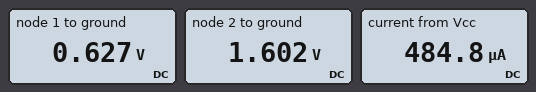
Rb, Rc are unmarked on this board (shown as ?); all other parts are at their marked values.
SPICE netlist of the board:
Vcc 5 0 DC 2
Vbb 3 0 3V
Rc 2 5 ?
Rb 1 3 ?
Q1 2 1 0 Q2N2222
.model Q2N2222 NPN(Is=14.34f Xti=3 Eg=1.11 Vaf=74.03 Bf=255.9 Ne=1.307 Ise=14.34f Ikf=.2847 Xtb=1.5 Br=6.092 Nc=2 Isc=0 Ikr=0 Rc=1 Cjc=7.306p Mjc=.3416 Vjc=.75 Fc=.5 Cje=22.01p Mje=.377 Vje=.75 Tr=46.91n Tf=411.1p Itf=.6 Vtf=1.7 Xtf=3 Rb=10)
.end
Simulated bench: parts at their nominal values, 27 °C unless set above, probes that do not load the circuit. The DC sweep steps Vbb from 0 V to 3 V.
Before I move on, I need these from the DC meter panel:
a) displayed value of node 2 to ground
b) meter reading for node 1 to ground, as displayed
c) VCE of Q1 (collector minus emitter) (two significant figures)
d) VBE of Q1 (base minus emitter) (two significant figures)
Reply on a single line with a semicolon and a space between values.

1.602 V; 0.627 V; 1.6 V; 630 mV
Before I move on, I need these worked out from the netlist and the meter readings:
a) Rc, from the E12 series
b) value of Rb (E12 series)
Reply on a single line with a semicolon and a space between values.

820 Ω; 680 kΩ
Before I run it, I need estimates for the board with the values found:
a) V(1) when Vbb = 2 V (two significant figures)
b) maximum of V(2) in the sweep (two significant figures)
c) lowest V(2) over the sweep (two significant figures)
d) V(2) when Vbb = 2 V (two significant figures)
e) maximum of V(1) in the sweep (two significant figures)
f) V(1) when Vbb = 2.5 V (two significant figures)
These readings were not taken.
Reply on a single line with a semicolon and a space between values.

610 mV; 2.0 V; 1.6 V; 1.8 V; 630 mV; 620 mV
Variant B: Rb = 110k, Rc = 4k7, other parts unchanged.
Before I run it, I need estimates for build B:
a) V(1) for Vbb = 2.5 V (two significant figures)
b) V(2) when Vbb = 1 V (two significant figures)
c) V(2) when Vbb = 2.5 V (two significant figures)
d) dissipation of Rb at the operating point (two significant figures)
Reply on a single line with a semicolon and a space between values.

630 mV; 130 mV; 48 mV; 51 µW
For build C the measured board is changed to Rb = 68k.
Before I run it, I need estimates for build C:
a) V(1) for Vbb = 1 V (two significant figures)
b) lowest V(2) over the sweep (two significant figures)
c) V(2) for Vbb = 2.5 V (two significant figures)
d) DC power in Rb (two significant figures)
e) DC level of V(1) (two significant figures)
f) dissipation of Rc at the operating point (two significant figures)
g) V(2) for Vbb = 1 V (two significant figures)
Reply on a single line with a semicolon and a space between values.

640 mV; 82 mV; 94 mV; 80 µW; 670 mV; 4.5 mW; 1.4 V
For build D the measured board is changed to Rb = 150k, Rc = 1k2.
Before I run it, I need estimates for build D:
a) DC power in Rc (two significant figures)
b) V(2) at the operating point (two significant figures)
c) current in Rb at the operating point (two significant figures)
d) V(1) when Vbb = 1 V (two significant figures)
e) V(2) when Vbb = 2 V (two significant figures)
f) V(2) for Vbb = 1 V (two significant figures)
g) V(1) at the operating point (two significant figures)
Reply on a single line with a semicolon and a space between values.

3.0 mW; 100 mV; 16 µA; 620 mV; 370 mV; 1.6 V; 660 mV
